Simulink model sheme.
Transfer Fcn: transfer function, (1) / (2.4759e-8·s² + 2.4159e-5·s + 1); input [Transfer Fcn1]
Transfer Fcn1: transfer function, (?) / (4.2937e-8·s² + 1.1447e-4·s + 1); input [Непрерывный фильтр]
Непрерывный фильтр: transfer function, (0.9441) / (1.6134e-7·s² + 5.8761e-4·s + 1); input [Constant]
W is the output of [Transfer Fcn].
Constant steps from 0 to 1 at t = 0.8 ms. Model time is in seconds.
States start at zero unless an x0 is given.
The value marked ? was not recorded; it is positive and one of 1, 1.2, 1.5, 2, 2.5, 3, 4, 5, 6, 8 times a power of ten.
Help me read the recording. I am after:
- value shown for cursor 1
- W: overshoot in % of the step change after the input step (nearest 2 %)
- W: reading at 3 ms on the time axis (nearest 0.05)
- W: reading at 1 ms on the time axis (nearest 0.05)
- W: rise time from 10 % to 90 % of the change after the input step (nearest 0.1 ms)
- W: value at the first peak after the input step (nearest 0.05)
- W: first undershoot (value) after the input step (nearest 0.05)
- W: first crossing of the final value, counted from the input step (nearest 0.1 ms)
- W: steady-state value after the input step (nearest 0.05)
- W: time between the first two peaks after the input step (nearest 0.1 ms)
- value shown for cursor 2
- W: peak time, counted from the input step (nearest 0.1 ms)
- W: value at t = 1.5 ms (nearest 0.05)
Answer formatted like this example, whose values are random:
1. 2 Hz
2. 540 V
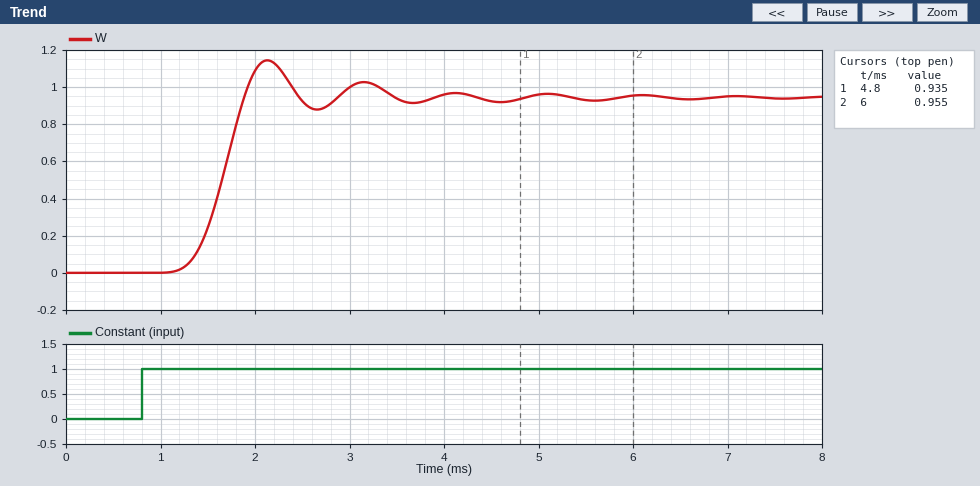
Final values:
1. 0.935
2. 22 %
3. 1.00
4. 0.00
5. 0.5 ms
6. 1.15
7. 0.90
8. 1.1 ms
9. 0.95
10. 1.0 ms
11. 0.955
12. 1.3 ms
13. 0.25
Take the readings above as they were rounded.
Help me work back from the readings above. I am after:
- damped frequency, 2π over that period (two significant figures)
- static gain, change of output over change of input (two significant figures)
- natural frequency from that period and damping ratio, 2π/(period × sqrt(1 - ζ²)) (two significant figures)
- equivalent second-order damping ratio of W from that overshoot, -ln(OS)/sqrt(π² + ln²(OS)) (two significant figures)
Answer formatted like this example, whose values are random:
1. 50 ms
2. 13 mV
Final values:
1. 6.3 rad/ms
2. 0.95
3. 7.0 rad/ms
4. 0.43
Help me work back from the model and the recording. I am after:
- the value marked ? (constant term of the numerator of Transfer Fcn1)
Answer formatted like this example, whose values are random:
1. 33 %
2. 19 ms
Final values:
1. 1
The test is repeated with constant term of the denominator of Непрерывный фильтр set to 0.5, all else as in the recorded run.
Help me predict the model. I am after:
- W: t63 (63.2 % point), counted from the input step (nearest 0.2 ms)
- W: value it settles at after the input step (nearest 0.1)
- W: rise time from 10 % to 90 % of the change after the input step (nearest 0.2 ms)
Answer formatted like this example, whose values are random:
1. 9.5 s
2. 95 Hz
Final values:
1. 1.2 ms
2. 1.9
3. 1.6 ms
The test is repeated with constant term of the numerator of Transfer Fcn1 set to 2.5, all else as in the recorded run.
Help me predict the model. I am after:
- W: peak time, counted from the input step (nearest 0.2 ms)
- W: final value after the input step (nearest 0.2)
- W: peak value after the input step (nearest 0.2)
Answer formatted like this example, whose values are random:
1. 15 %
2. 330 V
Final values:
1. 1.4 ms
2. 2.4
3. 2.8
